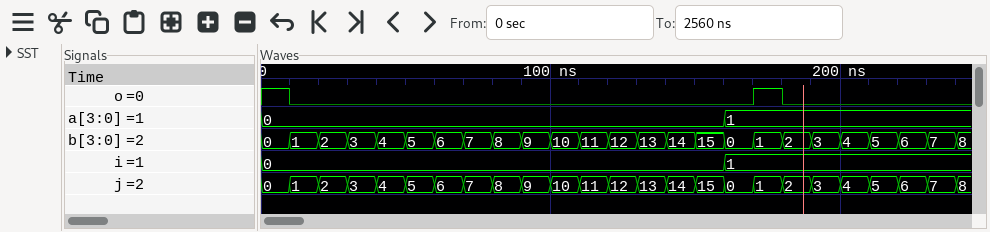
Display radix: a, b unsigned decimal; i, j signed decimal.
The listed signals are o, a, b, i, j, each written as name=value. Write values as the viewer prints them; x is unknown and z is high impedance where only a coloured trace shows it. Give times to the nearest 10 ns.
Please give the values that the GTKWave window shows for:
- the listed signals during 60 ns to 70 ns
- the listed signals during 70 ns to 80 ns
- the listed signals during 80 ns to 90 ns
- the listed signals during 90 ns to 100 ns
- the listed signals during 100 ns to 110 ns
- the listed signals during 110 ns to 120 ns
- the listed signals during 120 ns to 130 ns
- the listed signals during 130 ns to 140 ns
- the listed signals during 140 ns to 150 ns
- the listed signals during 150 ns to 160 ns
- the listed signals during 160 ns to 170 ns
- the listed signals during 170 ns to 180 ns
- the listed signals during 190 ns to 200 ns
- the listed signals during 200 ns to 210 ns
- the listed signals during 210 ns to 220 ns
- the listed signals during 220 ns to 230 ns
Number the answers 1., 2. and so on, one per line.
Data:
1. o=0, a=0, b=6, i=0, j=6
2. o=0, a=0, b=7, i=0, j=7
3. o=0, a=0, b=8, i=0, j=8
4. o=0, a=0, b=9, i=0, j=9
5. o=0, a=0, b=10, i=0, j=10
6. o=0, a=0, b=11, i=0, j=11
7. o=0, a=0, b=12, i=0, j=12
8. o=0, a=0, b=13, i=0, j=13
9. o=0, a=0, b=14, i=0, j=14
10. o=0, a=0, b=15, i=0, j=15
11. o=0, a=1, b=0, i=1, j=0
12. o=1, a=1, b=1, i=1, j=1
13. o=0, a=1, b=3, i=1, j=3
14. o=0, a=1, b=4, i=1, j=4
15. o=0, a=1, b=5, i=1, j=5
16. o=0, a=1, b=6, i=1, j=6
